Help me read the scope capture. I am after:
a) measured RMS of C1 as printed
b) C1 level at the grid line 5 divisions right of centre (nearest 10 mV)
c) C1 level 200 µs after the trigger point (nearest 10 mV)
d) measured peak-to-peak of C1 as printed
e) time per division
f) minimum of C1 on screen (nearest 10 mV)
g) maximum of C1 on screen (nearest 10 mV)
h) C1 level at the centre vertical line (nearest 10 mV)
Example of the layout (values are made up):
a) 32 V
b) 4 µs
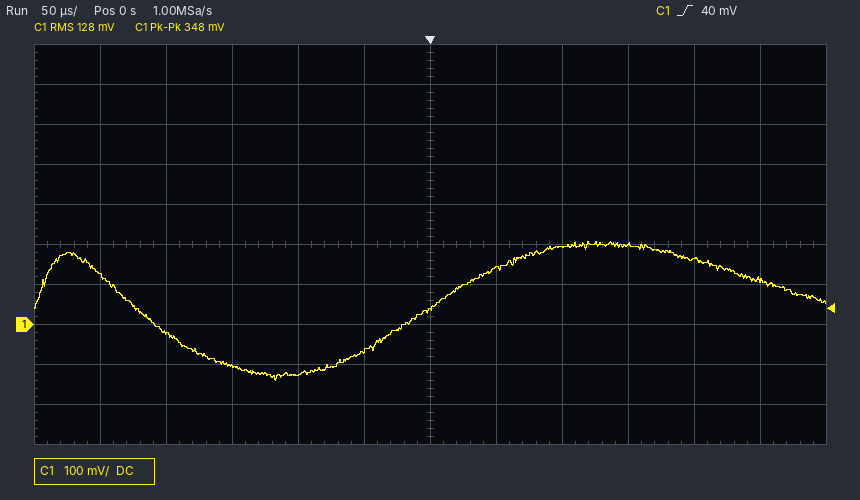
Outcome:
a) 128 mV
b) 110 mV
c) 160 mV
d) 348 mV
e) 50 µs
f) -140 mV
g) 210 mV
h) 40 mV
